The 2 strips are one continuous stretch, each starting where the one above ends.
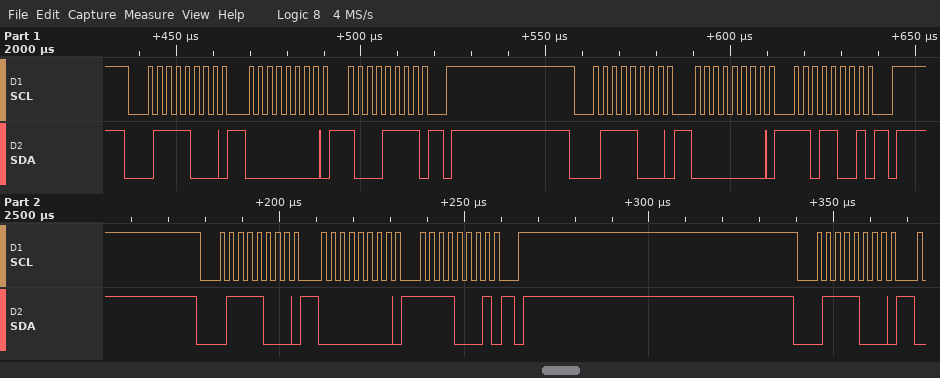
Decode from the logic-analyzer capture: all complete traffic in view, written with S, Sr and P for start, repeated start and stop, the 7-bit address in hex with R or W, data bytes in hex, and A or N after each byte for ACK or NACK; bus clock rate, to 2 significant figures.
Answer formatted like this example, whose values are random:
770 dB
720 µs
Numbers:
S 3CW A 00 A 8F A P S 3CW A 00 A D9 A P S 3CW A 00 A F1 A P S 3CW A
400 kHz
